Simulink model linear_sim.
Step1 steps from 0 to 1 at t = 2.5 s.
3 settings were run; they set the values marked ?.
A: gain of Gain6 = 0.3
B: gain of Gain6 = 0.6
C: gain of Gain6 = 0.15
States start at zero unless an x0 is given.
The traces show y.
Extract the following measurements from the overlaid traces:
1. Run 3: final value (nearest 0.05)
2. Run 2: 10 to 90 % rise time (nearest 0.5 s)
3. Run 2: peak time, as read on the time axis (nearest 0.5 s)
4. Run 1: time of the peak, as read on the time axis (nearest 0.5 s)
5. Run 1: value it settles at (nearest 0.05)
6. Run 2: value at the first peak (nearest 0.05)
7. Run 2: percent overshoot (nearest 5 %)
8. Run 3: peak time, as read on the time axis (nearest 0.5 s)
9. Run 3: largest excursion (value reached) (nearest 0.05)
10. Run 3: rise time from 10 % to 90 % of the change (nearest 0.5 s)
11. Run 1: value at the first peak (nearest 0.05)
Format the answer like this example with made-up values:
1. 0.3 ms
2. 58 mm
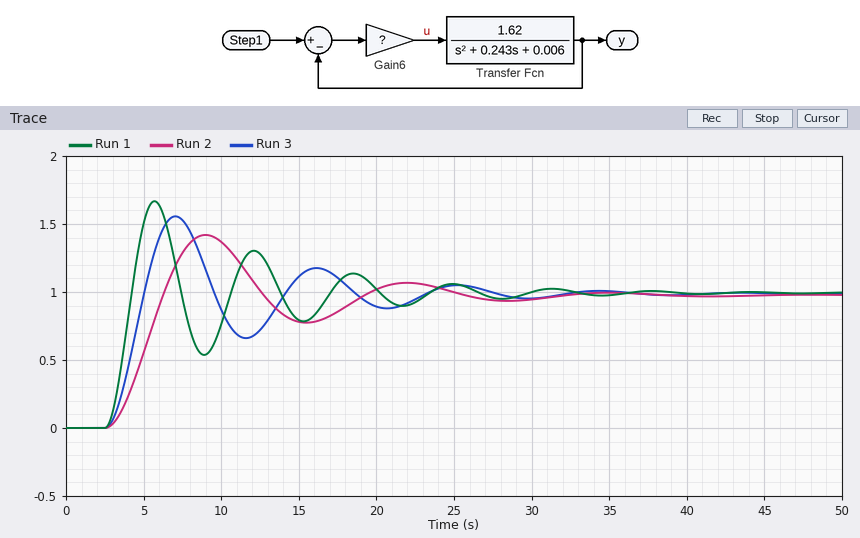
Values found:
1. 1.00
2. 2.5 s
3. 9.0 s
4. 5.5 s
5. 1.00
6. 1.40
7. 45 %
8. 7.0 s
9. 1.55
10. 1.5 s
11. 1.65
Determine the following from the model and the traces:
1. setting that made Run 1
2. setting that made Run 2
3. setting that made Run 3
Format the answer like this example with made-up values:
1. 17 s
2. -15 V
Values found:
1. B
2. C
3. A
